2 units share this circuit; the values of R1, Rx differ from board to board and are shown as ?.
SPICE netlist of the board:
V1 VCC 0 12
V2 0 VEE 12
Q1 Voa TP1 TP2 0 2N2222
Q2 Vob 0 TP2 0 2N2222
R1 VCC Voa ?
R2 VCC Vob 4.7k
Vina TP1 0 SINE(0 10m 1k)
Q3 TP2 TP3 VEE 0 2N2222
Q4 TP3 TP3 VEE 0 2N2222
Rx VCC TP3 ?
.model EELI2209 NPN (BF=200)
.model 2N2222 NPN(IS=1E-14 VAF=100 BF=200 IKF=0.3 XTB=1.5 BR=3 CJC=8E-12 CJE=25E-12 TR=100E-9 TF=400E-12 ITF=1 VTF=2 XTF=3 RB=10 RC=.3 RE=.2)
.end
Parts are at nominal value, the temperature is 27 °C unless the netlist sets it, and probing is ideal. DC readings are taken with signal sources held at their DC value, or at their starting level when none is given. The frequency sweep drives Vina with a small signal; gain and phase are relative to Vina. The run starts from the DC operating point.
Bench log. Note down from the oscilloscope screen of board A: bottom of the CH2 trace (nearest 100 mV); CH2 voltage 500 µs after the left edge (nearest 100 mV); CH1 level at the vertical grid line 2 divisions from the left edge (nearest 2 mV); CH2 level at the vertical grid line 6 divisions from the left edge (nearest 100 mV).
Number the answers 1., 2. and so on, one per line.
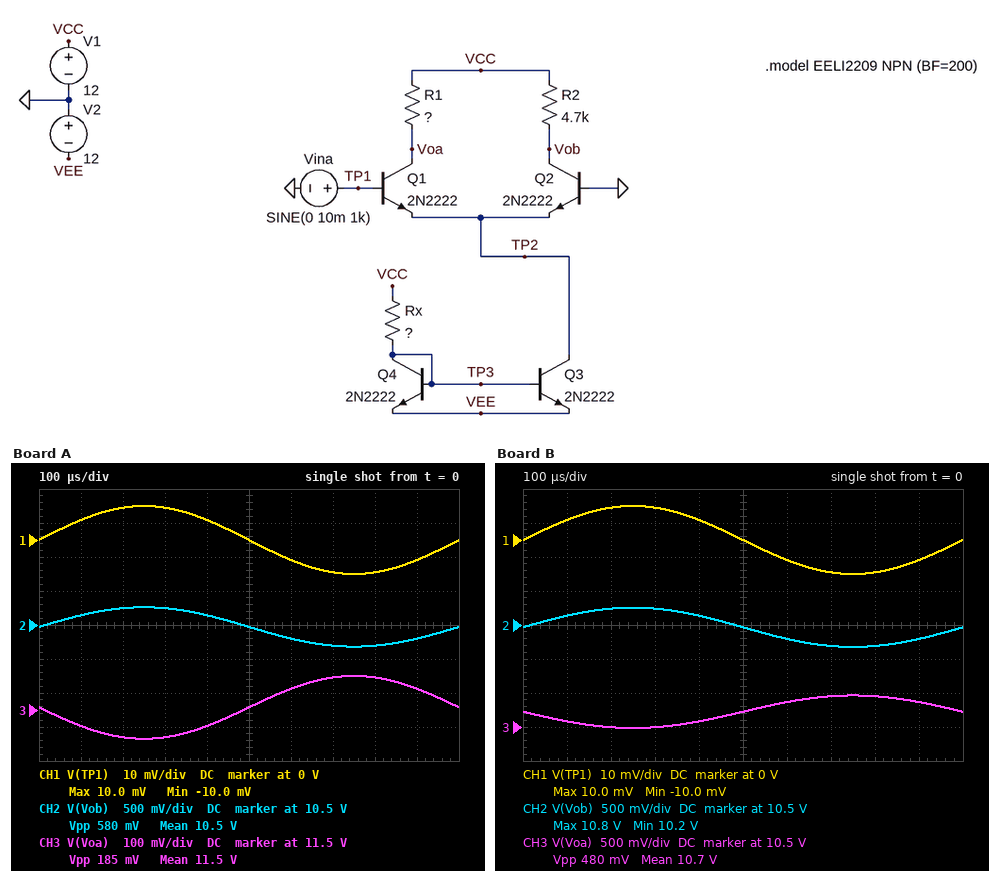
1. 10.2 V
2. 10.5 V
3. 10 mV
4. 10.3 V
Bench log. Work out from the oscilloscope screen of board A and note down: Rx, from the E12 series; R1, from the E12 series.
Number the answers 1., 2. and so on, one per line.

1. 39 kΩ
2. 1.5 kΩ
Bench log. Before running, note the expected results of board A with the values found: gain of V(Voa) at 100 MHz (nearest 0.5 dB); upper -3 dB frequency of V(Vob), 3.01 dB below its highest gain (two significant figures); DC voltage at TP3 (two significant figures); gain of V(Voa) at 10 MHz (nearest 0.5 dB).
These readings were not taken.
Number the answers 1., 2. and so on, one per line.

1. 9.5 dB
2. 9.5 MHz
3. -11 V
4. 19.0 dB
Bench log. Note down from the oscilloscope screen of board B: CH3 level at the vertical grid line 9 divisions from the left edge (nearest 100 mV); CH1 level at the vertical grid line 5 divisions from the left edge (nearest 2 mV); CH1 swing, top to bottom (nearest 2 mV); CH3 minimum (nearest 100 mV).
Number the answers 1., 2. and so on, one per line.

1. 10.9 V
2. 0 V
3. 20 mV
4. 10.5 V
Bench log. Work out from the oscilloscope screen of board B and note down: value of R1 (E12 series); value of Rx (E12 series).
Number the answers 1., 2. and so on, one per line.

1. 3.9 kΩ
2. 39 kΩ
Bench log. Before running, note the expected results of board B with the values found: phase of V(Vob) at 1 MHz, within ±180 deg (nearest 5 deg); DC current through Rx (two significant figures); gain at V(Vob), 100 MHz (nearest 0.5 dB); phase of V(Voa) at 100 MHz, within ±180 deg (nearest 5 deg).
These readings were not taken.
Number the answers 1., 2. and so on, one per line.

1. -5 deg
2. 600 µA
3. 7.5 dB
4. 65 deg
